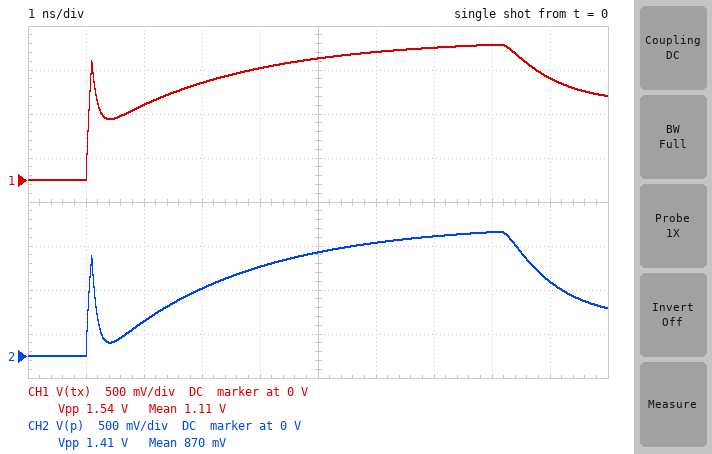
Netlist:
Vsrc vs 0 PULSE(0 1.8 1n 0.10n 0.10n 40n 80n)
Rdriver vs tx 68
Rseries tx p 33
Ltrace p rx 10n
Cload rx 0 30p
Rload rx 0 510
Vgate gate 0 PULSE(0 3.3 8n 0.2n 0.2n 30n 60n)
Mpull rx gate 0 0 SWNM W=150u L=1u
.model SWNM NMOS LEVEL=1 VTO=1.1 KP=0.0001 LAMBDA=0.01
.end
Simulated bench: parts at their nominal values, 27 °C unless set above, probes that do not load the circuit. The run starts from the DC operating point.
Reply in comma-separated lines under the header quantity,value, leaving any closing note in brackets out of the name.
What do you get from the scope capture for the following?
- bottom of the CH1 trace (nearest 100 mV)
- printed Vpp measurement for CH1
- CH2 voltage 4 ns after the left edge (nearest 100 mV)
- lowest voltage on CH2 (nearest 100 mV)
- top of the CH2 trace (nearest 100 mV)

quantity,value
bottom of the CH1 trace,0 V
printed Vpp measurement for CH1,1.54 V
CH2 voltage 4 ns after the left edge,1.0 V
lowest voltage on CH2,0 V
top of the CH2 trace,1.4 V
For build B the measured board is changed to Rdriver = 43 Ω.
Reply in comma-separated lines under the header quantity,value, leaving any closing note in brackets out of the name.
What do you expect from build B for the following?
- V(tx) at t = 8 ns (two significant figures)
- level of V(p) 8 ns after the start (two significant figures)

quantity,value
V(tx) at t = 8 ns,1.6 V
level of V(p) 8 ns after the start,1.5 V
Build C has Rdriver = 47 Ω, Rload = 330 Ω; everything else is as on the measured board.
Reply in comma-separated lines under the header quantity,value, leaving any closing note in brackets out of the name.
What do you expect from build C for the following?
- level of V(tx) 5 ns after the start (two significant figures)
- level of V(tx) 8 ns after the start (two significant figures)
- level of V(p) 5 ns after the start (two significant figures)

quantity,value
level of V(tx) 5 ns after the start,1.5 V
level of V(tx) 8 ns after the start,1.6 V
level of V(p) 5 ns after the start,1.3 V
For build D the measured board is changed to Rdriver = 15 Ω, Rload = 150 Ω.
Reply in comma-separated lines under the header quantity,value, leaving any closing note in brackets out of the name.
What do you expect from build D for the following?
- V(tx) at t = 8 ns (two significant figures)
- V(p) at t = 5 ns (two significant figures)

quantity,value
V(tx) at t = 8 ns,1.7 V
V(p) at t = 5 ns,1.3 V
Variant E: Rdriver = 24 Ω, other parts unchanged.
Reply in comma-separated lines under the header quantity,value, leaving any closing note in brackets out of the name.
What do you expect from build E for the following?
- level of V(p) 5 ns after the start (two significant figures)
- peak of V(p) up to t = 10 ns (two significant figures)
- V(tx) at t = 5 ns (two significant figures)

quantity,value
level of V(p) 5 ns after the start,1.5 V
peak of V(p) up to t = 10 ns,1.6 V
V(tx) at t = 5 ns,1.7 V
